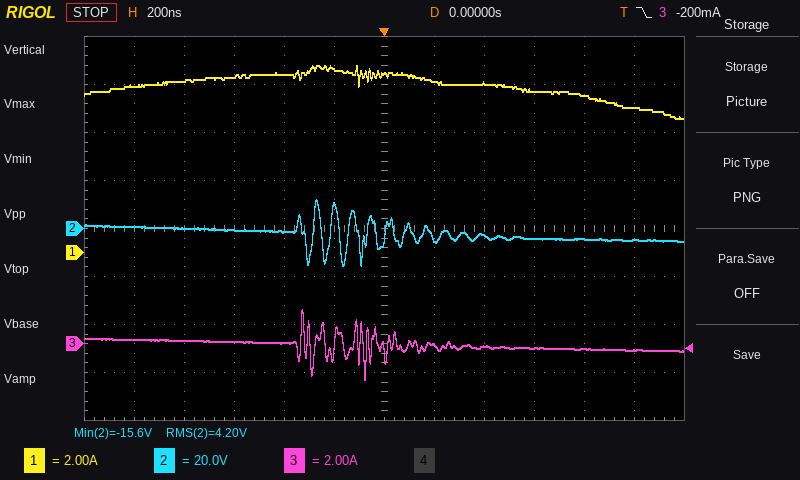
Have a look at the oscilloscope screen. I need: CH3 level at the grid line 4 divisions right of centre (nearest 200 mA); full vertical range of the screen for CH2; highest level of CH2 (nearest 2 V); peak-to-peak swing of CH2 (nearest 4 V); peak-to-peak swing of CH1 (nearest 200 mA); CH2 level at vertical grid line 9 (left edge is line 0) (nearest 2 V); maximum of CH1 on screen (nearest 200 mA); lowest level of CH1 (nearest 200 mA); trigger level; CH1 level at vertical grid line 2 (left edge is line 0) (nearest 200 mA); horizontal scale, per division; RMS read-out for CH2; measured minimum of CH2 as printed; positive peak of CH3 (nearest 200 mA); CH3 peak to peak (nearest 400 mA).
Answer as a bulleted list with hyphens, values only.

- -200 mA
- 160 V
- 12 V
- 28 V
- 2.2 A
- -4 V
- 7.8 A
- 5.6 A
- -200 mA
- 7.2 A
- 200 ns
- 4.20 V
- -15.6 V
- 1.4 A
- 2.8 A
